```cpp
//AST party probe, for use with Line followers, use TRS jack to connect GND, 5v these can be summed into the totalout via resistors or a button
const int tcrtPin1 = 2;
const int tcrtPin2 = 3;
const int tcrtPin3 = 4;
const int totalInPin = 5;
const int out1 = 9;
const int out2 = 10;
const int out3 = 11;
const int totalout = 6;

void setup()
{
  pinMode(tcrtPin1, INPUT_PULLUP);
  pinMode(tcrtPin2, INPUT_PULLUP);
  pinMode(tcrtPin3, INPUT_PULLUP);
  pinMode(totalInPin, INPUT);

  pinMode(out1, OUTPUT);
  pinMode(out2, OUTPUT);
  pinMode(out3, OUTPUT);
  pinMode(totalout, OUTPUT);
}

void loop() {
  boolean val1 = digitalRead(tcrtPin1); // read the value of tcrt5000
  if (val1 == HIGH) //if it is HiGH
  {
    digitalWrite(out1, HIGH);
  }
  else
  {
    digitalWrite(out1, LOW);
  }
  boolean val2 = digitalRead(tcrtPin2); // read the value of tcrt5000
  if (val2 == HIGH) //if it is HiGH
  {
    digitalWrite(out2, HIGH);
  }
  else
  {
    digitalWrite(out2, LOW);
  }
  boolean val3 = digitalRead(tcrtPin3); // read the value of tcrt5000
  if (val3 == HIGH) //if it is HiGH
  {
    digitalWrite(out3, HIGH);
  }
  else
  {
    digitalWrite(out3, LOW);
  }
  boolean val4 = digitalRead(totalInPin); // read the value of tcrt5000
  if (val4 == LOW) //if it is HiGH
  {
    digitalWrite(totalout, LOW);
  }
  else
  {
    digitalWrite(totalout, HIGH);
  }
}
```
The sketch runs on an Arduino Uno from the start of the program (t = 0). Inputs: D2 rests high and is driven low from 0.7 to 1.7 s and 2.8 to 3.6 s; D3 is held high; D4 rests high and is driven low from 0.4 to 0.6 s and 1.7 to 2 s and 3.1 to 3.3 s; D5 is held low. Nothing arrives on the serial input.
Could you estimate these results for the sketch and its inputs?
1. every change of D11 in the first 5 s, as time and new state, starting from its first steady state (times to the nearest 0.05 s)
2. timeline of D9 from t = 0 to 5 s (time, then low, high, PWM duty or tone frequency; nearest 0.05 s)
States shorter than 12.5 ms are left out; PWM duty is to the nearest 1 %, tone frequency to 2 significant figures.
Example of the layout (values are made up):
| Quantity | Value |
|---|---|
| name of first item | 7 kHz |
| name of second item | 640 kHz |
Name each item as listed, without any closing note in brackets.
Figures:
| Quantity | Value |
|---|---|
| every change of D11 in the first 5 s, as time and new state, starting from its first steady state | 0 s high; 0.4 s low; 0.6 s high; 1.7 s low; 2 s high; 3.1 s low; 3.3 s high |
| timeline of D9 from t = 0 to 5 s | 0 s high; 0.7 s low; 1.7 s high; 2.8 s low; 3.6 s high |
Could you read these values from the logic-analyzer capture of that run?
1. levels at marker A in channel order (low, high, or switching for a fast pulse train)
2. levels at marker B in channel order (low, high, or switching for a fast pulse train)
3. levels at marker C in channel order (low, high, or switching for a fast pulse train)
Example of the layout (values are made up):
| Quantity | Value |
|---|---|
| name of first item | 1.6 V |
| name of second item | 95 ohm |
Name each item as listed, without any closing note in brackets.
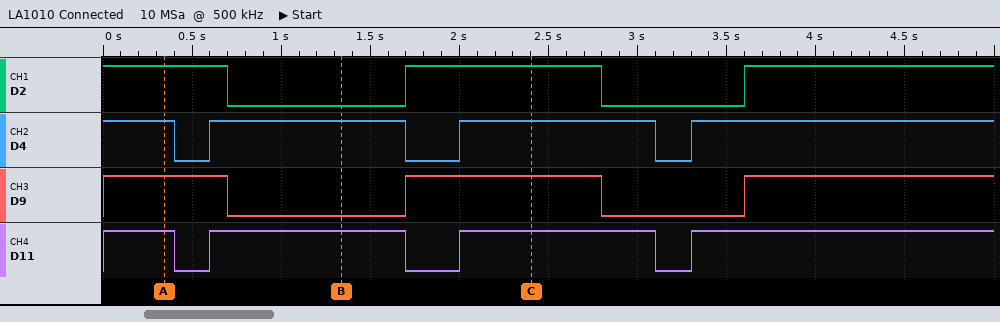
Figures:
| Quantity | Value |
|---|---|
| levels at marker A in channel order | D2 high, D4 high, D9 high, D11 high |
| levels at marker B in channel order | D2 low, D4 high, D9 low, D11 high |
| levels at marker C in channel order | D2 high, D4 high, D9 high, D11 high |
